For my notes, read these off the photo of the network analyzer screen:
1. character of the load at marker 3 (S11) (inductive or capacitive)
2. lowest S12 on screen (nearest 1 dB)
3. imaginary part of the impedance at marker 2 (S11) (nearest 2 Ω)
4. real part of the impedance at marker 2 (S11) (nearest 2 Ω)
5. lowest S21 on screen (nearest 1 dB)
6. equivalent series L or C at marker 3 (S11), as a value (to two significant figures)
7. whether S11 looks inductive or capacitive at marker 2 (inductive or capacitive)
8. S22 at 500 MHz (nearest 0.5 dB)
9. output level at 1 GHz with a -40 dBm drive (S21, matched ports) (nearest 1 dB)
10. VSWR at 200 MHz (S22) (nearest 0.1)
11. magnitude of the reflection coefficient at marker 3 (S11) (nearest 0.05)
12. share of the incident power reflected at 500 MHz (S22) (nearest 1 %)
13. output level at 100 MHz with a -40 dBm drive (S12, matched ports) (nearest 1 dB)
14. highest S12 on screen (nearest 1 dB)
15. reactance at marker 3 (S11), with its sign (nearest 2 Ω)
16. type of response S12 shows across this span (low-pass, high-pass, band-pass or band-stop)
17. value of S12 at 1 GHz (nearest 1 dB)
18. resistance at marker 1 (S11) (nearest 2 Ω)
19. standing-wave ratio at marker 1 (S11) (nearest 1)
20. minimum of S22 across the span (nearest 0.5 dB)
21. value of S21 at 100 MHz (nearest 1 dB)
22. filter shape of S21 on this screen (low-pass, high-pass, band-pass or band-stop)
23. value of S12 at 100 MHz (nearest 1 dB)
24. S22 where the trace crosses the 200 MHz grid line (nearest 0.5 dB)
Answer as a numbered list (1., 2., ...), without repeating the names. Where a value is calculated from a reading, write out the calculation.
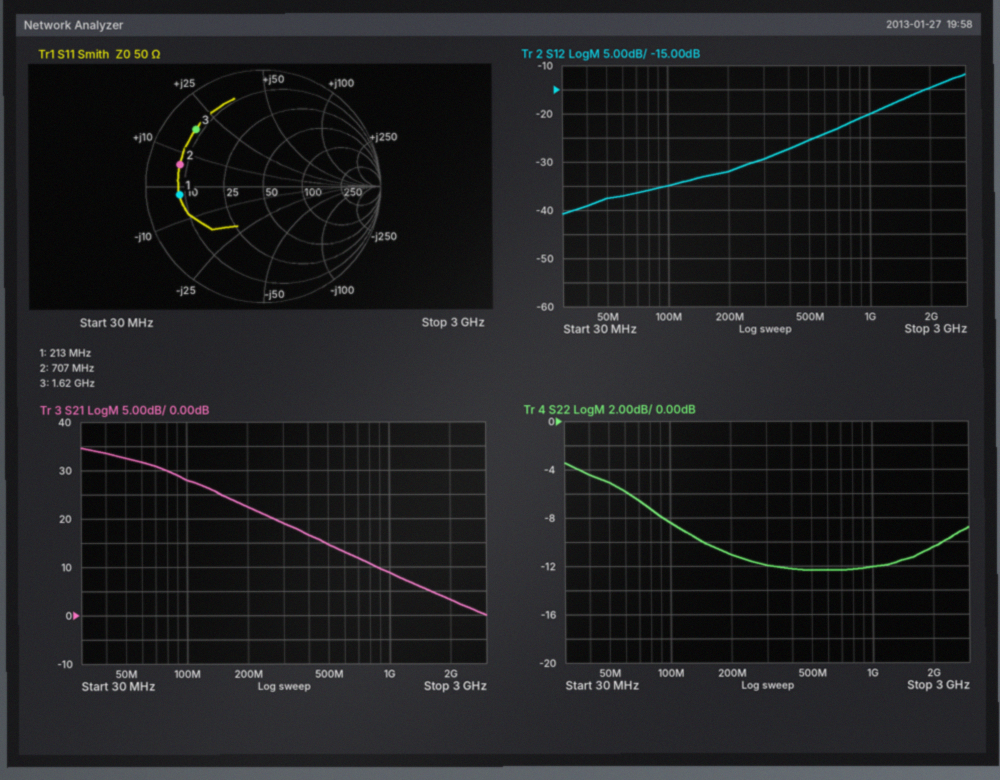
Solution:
1. inductive
2. -41 dB
3. +6 Ω
4. 8 Ω
5. 0 dB
6. L = 18 Ω/(2π × 1.62 GHz) ≈ 1.8 nH
7. inductive
8. -12.5 dB
9. -40 dBm + (9 dB) = -31 dBm
10. |Γ| = 10^(-11/20) = 0.2818; VSWR = (1 + 0.2818)/(1 − 0.2818) ≈ 1.8
11. 0.75
12. 10^(-12.5/10) ≈ 6 %
13. -40 dBm + (-35 dB) = -75 dBm
14. -12 dB
15. +18 Ω
16. high-pass
17. -20 dB
18. 8 Ω
19. 6
20. -12.5 dB
21. 28 dB
22. low-pass
23. -35 dB
24. -11.0 dB
